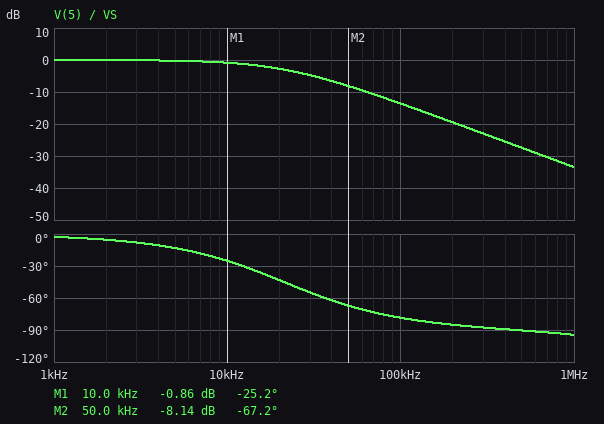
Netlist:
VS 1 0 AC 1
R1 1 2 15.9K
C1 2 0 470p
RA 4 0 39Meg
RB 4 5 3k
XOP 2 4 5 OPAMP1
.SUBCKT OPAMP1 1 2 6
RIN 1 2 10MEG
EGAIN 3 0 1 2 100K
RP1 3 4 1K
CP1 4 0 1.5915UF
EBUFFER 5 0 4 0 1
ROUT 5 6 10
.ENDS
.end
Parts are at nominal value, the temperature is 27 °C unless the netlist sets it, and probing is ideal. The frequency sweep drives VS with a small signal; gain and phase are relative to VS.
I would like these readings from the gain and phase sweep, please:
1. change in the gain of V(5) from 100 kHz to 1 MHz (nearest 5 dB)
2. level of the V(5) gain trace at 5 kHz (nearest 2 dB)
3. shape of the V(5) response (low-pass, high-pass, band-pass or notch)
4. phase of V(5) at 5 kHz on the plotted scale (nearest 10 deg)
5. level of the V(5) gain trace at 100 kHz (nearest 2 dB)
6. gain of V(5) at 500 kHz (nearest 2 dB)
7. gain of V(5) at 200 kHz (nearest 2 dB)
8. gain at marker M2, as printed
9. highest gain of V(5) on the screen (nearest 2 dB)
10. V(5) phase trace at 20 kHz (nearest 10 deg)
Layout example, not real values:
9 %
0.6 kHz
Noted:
-20 dB
0 dB
low-pass
-10 deg
-14 dB
-28 dB
-20 dB
-8.14 dB
0 dB
-40 deg
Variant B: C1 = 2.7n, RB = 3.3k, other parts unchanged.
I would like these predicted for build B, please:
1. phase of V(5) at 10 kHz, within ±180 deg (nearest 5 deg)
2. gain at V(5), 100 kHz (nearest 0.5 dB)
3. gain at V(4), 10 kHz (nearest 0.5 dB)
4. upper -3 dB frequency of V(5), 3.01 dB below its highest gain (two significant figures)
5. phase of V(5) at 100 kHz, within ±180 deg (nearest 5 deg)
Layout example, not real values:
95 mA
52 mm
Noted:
-70 deg
-28.5 dB
-9.0 dB
3.7 kHz
-90 deg
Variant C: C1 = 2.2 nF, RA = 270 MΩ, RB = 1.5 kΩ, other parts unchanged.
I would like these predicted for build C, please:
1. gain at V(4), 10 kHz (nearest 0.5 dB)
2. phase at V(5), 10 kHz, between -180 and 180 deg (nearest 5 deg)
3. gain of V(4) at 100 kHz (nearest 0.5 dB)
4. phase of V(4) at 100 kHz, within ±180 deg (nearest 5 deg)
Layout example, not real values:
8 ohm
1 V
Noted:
-7.5 dB
-65 deg
-27.0 dB
-90 deg
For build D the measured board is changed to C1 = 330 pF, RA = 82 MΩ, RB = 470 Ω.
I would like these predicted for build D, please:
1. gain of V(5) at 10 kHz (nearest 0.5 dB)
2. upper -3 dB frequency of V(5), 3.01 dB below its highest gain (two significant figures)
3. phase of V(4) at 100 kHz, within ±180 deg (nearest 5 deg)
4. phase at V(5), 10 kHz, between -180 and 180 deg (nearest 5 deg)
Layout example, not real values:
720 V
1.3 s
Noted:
-0.5 dB
30 kHz
-75 deg
-20 deg
